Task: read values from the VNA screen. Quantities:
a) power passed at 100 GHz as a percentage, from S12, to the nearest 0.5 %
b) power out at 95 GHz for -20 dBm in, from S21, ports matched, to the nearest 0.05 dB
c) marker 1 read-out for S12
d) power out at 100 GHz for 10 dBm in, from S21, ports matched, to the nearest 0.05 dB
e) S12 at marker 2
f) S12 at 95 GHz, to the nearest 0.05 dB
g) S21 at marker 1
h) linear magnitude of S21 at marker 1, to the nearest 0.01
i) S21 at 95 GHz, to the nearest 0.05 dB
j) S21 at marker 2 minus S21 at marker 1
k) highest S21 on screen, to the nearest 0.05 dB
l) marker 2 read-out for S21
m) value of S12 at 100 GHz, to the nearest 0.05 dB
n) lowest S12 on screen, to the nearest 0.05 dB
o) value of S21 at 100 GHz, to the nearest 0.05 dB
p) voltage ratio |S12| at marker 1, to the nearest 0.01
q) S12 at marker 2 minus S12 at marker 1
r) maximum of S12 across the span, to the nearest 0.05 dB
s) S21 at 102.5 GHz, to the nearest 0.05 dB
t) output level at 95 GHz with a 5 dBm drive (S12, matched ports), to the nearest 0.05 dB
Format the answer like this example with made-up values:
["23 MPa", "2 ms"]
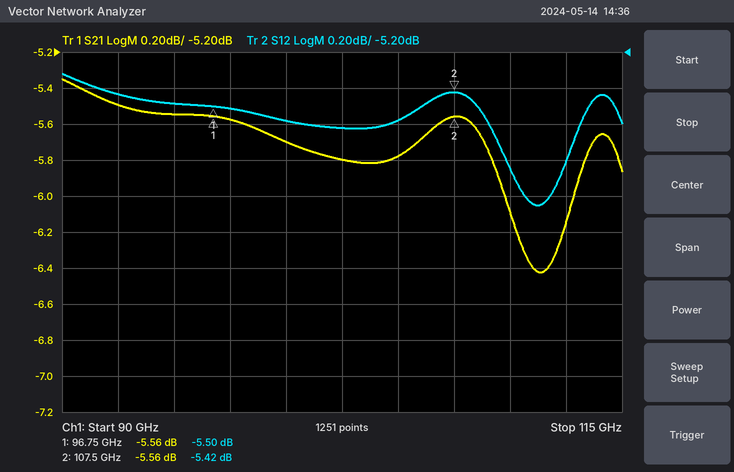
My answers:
["27.5 %", "-25.55 dBm", "-5.50 dB", "4.30 dBm", "-5.42 dB", "-5.50 dB", "-5.56 dB", "0.53", "-5.55 dB", "0.00 dB", "-5.35 dB", "-5.56 dB", "-5.60 dB", "-6.05 dB", "-5.70 dB", "0.53", "0.08 dB", "-5.30 dB", "-5.80 dB", "-0.50 dBm"]
